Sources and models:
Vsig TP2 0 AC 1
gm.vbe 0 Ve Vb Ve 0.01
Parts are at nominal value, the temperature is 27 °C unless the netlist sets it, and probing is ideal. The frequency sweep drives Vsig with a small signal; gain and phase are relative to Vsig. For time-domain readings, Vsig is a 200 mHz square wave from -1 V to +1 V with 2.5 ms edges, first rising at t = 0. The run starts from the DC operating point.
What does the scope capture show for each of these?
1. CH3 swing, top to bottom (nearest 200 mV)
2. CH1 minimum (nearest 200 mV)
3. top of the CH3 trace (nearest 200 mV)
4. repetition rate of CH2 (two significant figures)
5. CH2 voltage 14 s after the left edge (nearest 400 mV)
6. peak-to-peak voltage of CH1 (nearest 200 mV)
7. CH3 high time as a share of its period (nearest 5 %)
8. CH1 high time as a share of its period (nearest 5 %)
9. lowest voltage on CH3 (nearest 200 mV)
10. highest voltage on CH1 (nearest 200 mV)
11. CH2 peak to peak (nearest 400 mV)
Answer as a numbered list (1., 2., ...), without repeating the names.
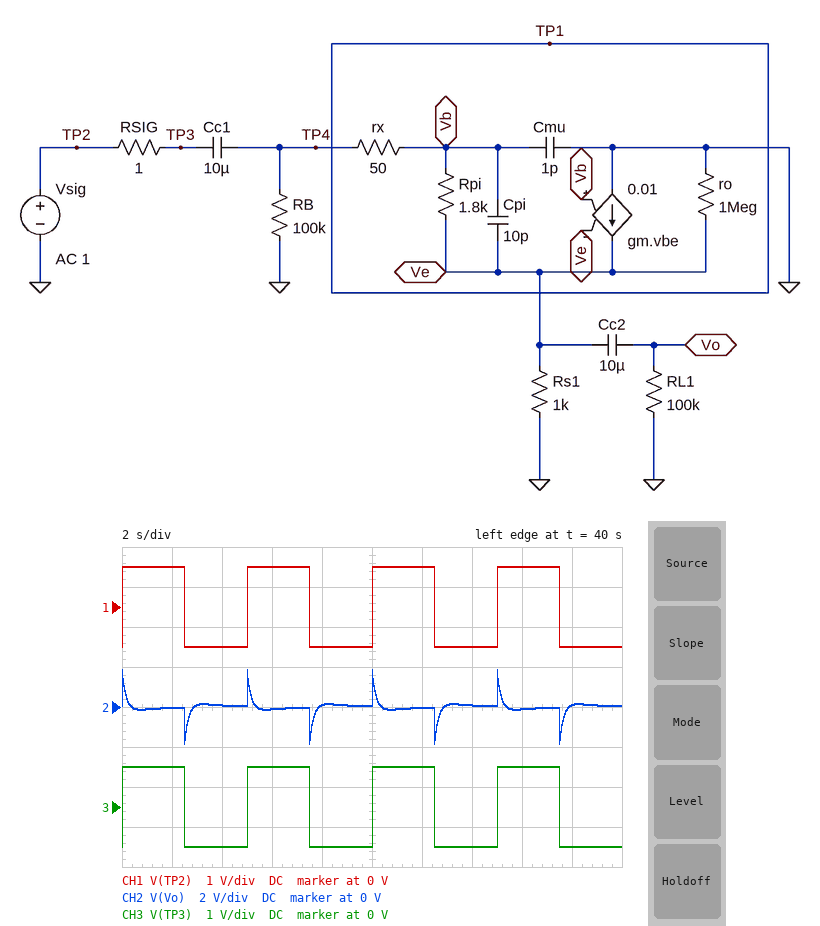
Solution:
1. 2.0 V
2. -1.0 V
3. 1.0 V
4. 200 mHz
5. 0 V
6. 2.0 V
7. 50 %
8. 50 %
9. -1.0 V
10. 1.0 V
11. 3.6 V
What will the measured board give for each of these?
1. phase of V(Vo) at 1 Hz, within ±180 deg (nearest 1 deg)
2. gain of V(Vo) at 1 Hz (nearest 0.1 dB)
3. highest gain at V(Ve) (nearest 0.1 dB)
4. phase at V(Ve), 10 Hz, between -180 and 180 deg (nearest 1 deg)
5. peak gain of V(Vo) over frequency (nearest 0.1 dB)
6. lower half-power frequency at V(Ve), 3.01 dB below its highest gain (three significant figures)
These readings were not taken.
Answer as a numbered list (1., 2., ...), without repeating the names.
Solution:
1. 52 deg
2. -3.6 dB
3. -0.8 dB
4. 5 deg
5. -0.8 dB
6. 931 mHz
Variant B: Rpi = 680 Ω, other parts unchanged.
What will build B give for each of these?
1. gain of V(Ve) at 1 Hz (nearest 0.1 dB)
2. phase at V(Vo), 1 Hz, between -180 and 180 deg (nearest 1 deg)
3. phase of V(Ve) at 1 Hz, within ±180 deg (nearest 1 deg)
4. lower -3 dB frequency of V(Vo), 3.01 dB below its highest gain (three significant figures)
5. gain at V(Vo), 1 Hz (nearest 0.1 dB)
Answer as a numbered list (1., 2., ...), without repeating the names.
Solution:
1. -7.9 dB
2. 73 deg
3. 64 deg
4. 2.06 Hz
5. -8.0 dB
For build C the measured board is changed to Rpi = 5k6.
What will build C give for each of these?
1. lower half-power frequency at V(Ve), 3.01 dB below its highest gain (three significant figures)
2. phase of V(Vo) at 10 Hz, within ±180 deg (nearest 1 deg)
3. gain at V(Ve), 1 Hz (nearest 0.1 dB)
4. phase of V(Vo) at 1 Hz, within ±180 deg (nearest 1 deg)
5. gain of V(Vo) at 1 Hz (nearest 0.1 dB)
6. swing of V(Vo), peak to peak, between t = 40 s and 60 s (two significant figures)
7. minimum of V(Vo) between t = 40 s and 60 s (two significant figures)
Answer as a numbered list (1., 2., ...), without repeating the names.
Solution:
1. 416 mHz
2. 3 deg
3. -1.5 dB
4. 32 deg
5. -1.6 dB
6. 3.8 V
7. -1.9 V
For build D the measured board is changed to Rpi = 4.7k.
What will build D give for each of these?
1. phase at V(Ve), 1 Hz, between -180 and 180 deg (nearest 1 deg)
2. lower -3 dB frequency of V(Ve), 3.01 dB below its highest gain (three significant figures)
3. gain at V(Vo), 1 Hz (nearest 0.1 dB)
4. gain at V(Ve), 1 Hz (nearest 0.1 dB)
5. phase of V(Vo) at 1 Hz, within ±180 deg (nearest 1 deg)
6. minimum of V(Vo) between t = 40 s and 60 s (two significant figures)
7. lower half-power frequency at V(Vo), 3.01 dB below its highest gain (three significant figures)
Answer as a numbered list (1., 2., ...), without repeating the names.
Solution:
1. 25 deg
2. 464 mHz
3. -1.8 dB
4. -1.7 dB
5. 34 deg
6. -1.9 V
7. 512 mHz
